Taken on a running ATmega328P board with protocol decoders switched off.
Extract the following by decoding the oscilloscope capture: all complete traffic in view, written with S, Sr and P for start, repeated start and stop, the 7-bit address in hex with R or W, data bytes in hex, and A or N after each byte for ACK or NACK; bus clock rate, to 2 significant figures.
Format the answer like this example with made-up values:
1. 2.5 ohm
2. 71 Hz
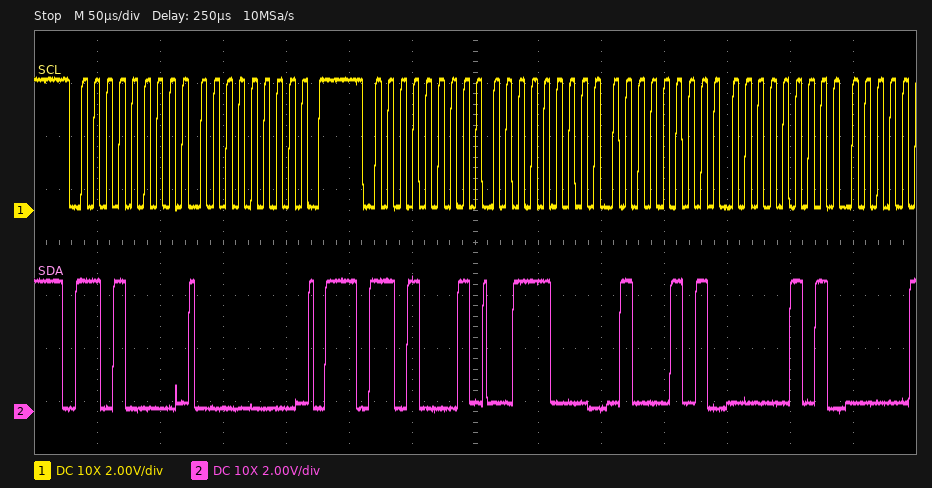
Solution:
1. S 68W A 00 A P S 68R A 38 A 45 A 05 A
2. 100 kHz
